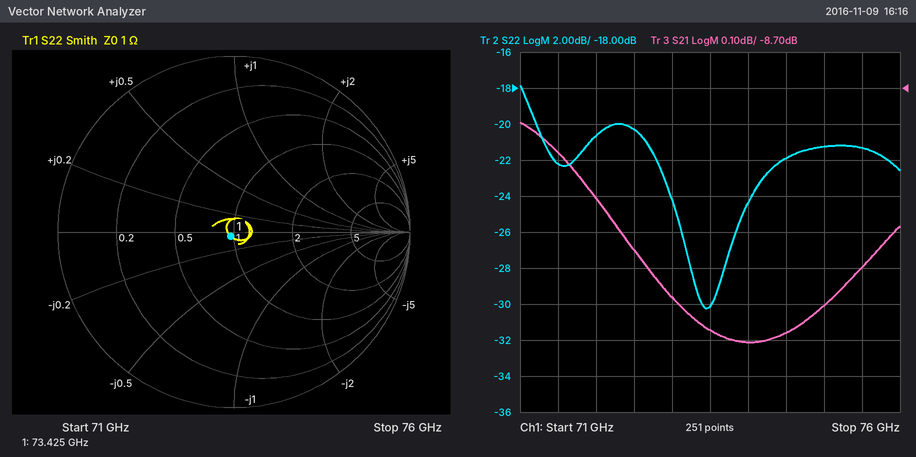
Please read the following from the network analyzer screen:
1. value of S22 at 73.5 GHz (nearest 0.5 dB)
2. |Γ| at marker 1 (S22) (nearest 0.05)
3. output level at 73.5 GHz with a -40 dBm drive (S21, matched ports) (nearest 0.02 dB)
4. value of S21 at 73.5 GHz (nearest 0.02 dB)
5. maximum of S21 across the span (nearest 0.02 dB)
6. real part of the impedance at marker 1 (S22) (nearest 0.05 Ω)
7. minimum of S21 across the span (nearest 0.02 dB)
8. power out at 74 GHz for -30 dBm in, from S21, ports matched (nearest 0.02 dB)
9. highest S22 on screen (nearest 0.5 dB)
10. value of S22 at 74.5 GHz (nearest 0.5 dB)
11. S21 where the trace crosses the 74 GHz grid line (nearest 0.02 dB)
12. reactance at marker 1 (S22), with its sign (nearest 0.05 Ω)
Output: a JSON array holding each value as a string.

["-30.0 dB", "0.05", "-49.38 dBm", "-9.38 dB", "-8.80 dB", "0.95 Ω", "-9.40 dB", "-39.40 dBm", "-18.0 dB", "-22.0 dB", "-9.40 dB", "-0.05 Ω"]
